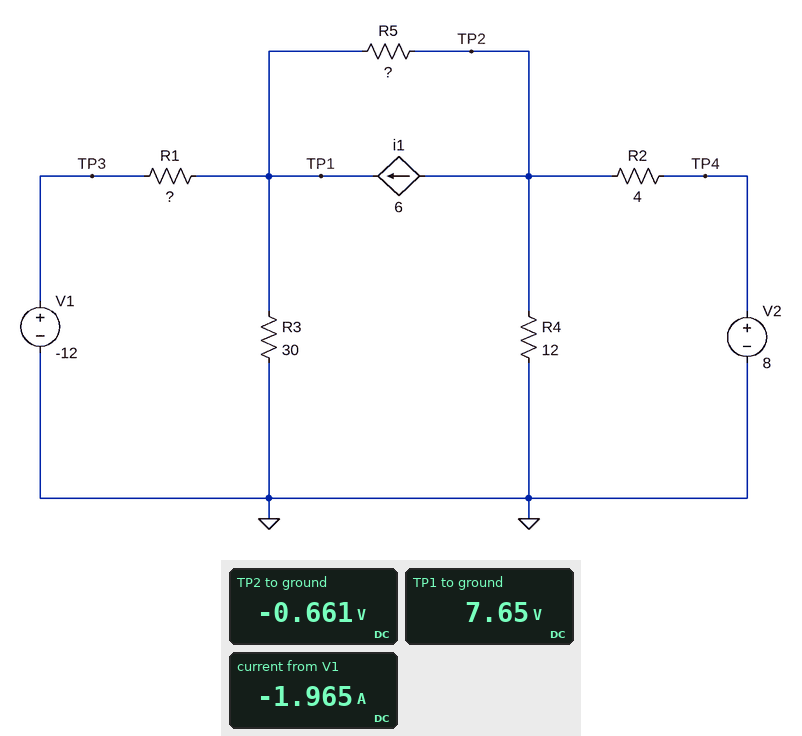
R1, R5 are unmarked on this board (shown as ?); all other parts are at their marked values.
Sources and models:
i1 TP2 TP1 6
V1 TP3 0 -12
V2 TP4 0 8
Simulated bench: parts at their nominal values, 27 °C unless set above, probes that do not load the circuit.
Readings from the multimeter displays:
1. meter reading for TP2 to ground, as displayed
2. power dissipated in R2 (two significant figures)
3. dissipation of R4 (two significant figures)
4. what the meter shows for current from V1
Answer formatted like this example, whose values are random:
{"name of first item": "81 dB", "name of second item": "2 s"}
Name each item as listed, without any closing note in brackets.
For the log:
{"meter reading for TP2 to ground, as displayed": "-0.661 V", "power dissipated in R2": "19 W", "dissipation of R4": "36 mW", "what the meter shows for current from V1": "-1.965 A"}
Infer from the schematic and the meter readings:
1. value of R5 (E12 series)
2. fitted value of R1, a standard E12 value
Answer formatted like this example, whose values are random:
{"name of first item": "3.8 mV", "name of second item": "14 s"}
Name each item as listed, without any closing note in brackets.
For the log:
{"value of R5": "2.2 Ω", "fitted value of R1, a standard E12 value": "10 Ω"}
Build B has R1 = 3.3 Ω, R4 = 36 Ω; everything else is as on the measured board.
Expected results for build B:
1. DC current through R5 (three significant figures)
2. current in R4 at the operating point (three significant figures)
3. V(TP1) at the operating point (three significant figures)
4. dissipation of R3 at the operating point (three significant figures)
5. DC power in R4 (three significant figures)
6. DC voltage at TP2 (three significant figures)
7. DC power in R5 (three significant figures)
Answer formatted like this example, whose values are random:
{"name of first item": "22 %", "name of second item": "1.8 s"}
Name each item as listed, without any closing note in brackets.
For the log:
{"DC current through R5": "2.44 A", "current in R4 at the operating point": "156 mA", "V(TP1) at the operating point": "-234 mV", "dissipation of R3 at the operating point": "1.83 mW", "DC power in R4": "873 mW", "DC voltage at TP2": "-5.61 V", "DC power in R5": "13.1 W"}
